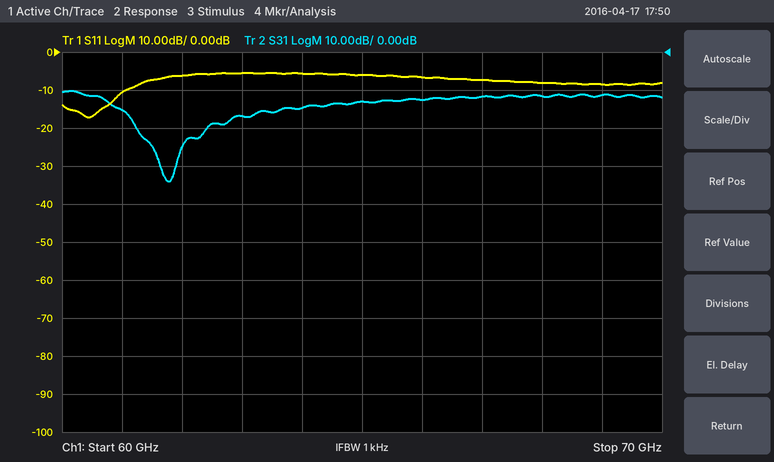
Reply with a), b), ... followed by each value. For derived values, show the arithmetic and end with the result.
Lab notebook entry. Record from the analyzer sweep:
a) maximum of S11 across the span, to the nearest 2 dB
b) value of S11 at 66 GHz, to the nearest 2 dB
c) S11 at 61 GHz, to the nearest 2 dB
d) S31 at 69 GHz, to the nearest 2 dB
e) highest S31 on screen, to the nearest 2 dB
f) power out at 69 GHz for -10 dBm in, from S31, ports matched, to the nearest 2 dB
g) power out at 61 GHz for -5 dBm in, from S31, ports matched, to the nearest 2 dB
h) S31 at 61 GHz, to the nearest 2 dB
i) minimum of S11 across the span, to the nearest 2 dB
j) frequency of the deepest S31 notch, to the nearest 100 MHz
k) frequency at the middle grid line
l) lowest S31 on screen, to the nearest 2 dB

a) -6 dB
b) -6 dB
c) -10 dB
d) -12 dB
e) -10 dB
f) -10 dBm + (-12 dB) = -22 dBm
g) -5 dBm + (-16 dB) = -20 dBm
h) -16 dB
i) -18 dB
j) 61.8 GHz
k) 65 GHz
l) -34 dB
